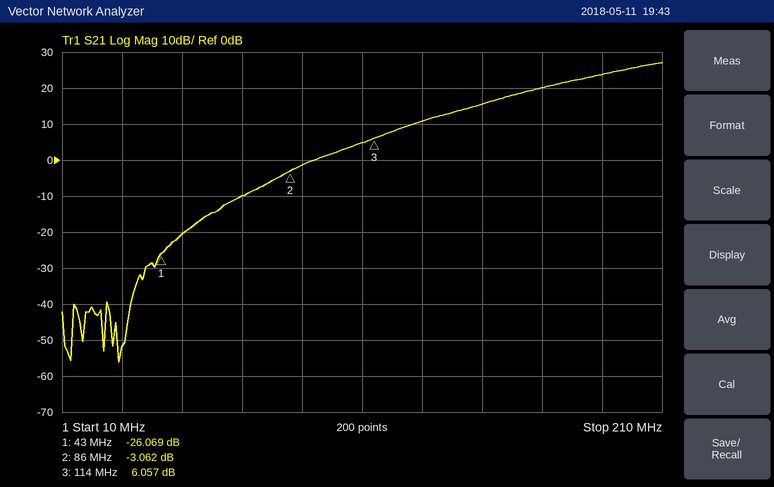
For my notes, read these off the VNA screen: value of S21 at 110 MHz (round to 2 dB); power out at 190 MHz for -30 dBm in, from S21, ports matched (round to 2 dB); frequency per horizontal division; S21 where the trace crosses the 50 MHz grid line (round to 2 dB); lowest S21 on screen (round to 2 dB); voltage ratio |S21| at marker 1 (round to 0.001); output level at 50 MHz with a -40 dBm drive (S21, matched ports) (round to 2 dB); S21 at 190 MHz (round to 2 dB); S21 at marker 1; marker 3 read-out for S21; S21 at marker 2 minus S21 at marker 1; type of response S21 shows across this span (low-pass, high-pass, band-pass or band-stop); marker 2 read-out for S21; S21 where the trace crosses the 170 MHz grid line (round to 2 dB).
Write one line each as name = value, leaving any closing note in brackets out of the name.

value of S21 at 110 MHz = 4 dB
power out at 190 MHz for -30 dBm in, from S21, ports matched = -6 dBm
frequency per horizontal division = 20 MHz
S21 where the trace crosses the 50 MHz grid line = -20 dB
lowest S21 on screen = -56 dB
voltage ratio |S21| at marker 1 = 0.050
output level at 50 MHz with a -40 dBm drive (S21, matched ports) = -60 dBm
S21 at 190 MHz = 24 dB
S21 at marker 1 = -26.069 dB
marker 3 read-out for S21 = 6.057 dB
S21 at marker 2 minus S21 at marker 1 = 23.007 dB
type of response S21 shows across this span = high-pass
marker 2 read-out for S21 = -3.062 dB
S21 where the trace crosses the 170 MHz grid line = 20 dB
